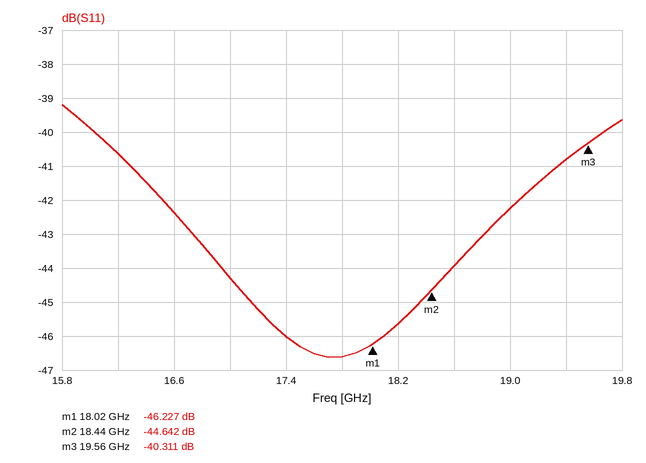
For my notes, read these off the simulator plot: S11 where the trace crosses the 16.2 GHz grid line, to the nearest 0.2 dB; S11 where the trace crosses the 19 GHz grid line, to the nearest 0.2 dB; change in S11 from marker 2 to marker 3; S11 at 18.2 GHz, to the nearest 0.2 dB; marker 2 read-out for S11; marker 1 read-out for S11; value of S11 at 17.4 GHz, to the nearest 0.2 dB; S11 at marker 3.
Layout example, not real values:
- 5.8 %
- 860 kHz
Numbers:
- -40.6 dB
- -42.2 dB
- 4.331 dB
- -45.6 dB
- -44.642 dB
- -46.227 dB
- -46.0 dB
- -40.311 dB
